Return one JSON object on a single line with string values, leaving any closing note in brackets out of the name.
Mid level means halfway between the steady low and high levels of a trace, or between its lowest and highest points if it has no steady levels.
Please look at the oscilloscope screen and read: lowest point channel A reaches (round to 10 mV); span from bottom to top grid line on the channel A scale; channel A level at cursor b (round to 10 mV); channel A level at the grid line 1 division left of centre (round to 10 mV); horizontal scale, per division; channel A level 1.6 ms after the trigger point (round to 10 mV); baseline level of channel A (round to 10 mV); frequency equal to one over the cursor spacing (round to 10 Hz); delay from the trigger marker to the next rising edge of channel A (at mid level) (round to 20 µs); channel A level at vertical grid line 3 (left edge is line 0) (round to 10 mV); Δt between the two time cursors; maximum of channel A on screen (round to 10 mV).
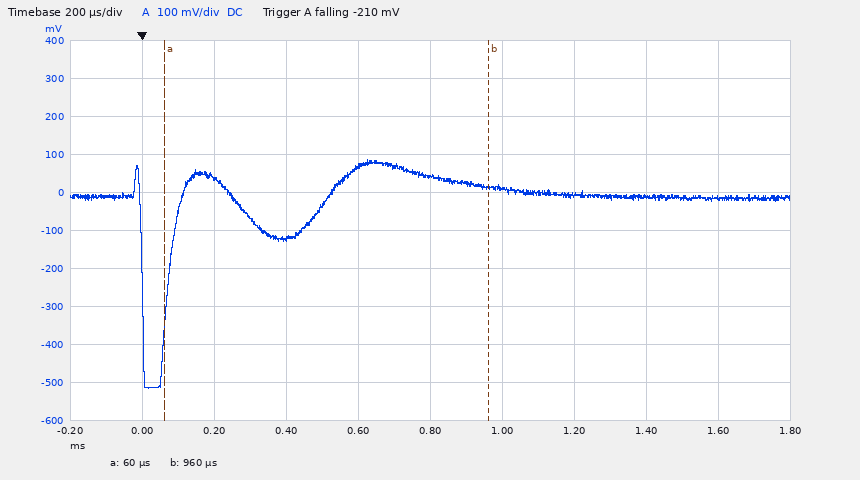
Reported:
{"lowest point channel A reaches": "-520 mV", "span from bottom to top grid line on the channel A scale": "1 V", "channel A level at cursor b": "10 mV", "channel A level at the grid line 1 division left of centre": "70 mV", "horizontal scale, per division": "200 µs", "channel A level 1.6 ms after the trigger point": "-10 mV", "baseline level of channel A": "-10 mV", "frequency equal to one over the cursor spacing": "1.11 kHz", "delay from the trigger marker to the next rising edge of channel A (at mid level)": "80 µs", "channel A level at vertical grid line 3 (left edge is line 0)": "-120 mV", "Δt between the two time cursors": "900 µs", "maximum of channel A on screen": "90 mV"}
